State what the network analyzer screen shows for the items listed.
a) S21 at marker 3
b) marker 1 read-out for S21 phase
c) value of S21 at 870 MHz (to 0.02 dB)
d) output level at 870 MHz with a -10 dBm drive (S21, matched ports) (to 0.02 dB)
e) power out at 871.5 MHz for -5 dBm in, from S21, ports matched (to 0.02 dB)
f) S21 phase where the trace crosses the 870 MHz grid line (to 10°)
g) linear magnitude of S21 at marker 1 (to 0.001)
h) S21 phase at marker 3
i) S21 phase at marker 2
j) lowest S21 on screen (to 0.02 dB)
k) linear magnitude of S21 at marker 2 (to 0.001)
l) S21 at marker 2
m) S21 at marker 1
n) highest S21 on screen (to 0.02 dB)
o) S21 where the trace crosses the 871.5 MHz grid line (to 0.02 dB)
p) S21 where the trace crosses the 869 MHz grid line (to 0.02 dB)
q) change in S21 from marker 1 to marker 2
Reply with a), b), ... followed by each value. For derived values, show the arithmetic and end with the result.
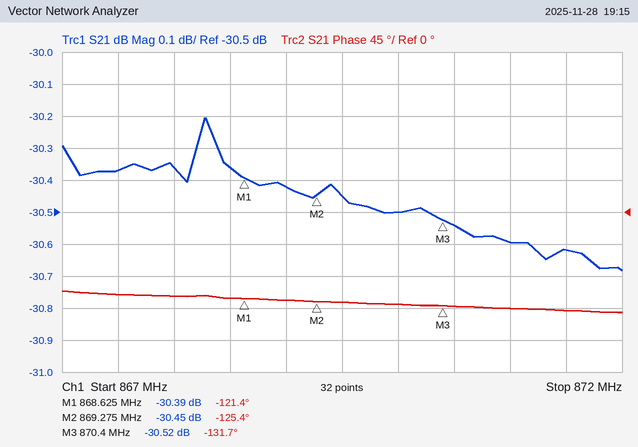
a) -30.52 dB
b) -121.4°
c) -30.50 dB
d) -10 dBm + (-30.50 dB) = -40.50 dBm
e) -5 dBm + (-30.62 dB) = -35.62 dBm
f) -130°
g) 10^(-30.39/20) ≈ 0.030
h) -131.7°
i) -125.4°
j) -30.68 dB
k) 10^(-30.45/20) ≈ 0.030
l) -30.45 dB
m) -30.39 dB
n) -30.20 dB
o) -30.62 dB
p) -30.42 dB
q) -30.45 − (-30.39) = -0.06 dB
